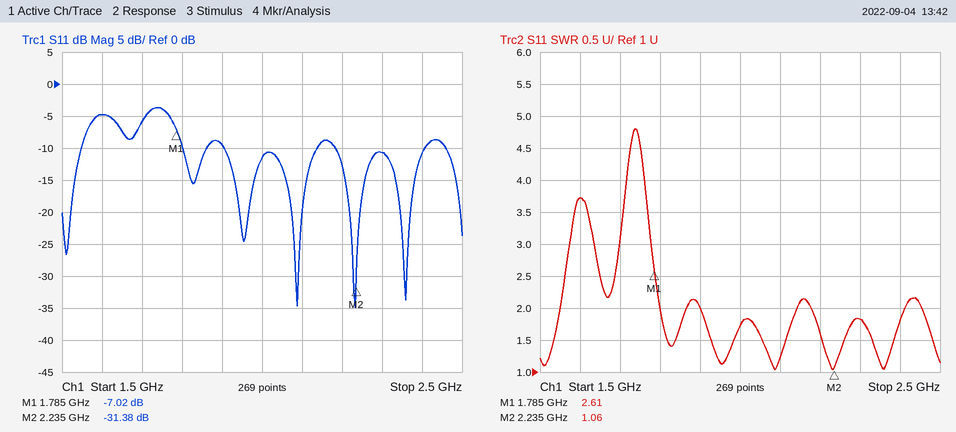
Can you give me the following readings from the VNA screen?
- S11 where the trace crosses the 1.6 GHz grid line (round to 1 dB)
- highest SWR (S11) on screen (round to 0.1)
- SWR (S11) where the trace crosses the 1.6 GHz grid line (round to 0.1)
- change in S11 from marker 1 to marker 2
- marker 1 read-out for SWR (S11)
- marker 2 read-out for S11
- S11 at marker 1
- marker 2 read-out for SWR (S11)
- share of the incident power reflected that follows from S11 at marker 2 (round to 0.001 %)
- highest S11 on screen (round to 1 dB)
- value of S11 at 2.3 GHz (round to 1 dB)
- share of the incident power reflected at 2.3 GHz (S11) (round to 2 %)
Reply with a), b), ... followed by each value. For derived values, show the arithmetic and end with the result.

a) -5 dB
b) 4.8
c) 3.7
d) -31.38 − (-7.02) = -24.36 dB
e) 2.61
f) -31.38 dB
g) -7.02 dB
h) 1.06
i) 10^(-31.38/10) ≈ 0.073 %
j) -4 dB
k) -11 dB
l) 10^(-11/10) ≈ 8 %
